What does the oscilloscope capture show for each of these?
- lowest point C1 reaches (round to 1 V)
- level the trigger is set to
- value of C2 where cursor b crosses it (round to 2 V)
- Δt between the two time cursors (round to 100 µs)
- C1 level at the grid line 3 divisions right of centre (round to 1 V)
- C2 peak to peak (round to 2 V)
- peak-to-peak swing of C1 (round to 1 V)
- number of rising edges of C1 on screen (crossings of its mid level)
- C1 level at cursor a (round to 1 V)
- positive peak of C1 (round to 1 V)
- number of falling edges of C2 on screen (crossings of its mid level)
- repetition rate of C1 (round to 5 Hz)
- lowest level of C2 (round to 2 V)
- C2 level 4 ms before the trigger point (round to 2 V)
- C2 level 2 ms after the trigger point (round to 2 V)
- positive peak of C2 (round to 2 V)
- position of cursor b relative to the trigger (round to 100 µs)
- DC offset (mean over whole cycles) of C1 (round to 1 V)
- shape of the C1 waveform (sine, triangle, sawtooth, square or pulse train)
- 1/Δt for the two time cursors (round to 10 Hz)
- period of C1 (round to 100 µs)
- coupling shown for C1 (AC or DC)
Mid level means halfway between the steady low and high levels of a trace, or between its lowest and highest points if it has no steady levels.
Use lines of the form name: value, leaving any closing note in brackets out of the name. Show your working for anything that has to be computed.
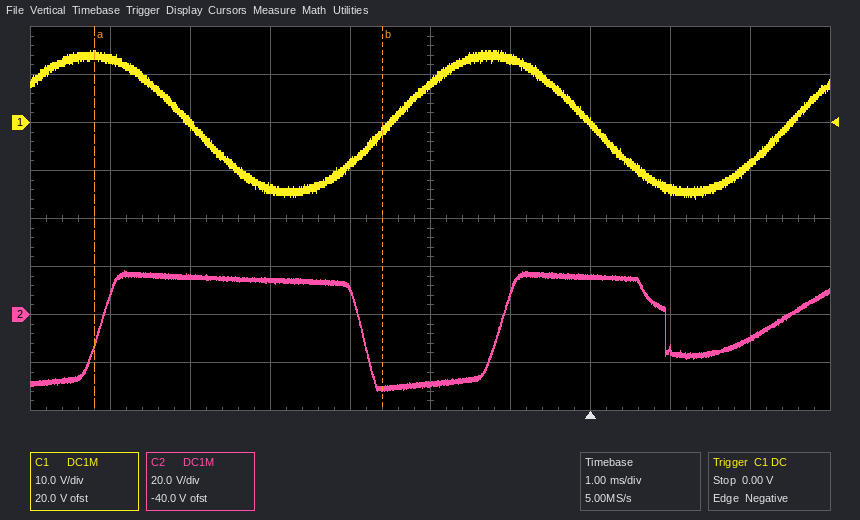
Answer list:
lowest point C1 reaches: -16 V
level the trigger is set to: 0.00 V
value of C2 where cursor b crosses it: -30 V
Δt between the two time cursors: 3.6 ms
C1 level at the grid line 3 divisions right of centre: -14 V
C2 peak to peak: 18 V − (-32 V) = 50 V
peak-to-peak swing of C1: 15 V − (-16 V) = 31 V
number of rising edges of C1 on screen: 2
C1 level at cursor a: 14 V
positive peak of C1: 15 V
number of falling edges of C2 on screen: 2
repetition rate of C1: 1 / 5.0 ms ≈ 200 Hz
lowest level of C2: -32 V
C2 level 4 ms before the trigger point: 14 V
C2 level 2 ms after the trigger point: -10 V
positive peak of C2: 18 V
position of cursor b relative to the trigger: -2.6 ms
DC offset (mean over whole cycles) of C1: (15 V + (-16 V)) / 2 ≈ 0 V
shape of the C1 waveform: sine
1/Δt for the two time cursors: 1 / 3.6 ms ≈ 280 Hz
period of C1: 5.0 ms
coupling shown for C1: DC
